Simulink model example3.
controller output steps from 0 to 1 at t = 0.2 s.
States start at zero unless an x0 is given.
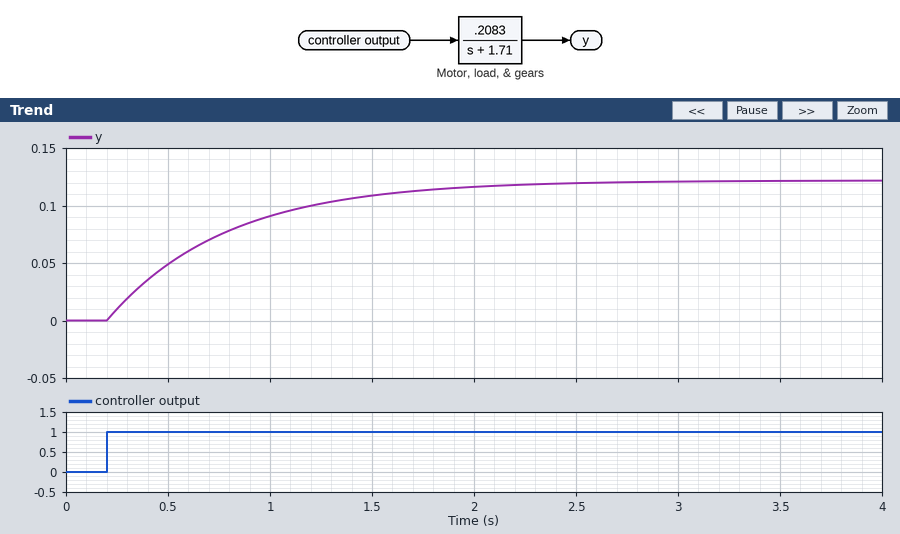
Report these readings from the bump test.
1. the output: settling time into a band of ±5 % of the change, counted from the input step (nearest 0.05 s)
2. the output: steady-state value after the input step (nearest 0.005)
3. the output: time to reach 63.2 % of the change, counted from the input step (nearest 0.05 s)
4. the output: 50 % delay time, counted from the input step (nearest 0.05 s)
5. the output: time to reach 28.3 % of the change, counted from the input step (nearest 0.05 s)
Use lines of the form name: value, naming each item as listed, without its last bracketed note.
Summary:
the output: settling time into a band of ±5 % of the change, counted from the input step: 1.75 s
the output: steady-state value after the input step: 0.120
the output: time to reach 63.2 % of the change, counted from the input step: 0.60 s
the output: 50 % delay time, counted from the input step: 0.40 s
the output: time to reach 28.3 % of the change, counted from the input step: 0.20 s
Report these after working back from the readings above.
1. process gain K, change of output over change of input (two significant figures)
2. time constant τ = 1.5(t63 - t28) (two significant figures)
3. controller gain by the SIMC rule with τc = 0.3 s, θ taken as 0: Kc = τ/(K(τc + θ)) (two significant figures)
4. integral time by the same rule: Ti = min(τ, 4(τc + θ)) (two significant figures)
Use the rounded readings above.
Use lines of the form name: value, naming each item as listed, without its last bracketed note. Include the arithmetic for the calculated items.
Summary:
process gain K, change of output over change of input: (0.12 - 0) / 1 = 0.12
time constant τ = 1.5(t63 - t28): 1.5 × (0.6 - 0.2) = 0.60 s
controller gain by the SIMC rule with τc = 0.3 s, θ taken as 0: Kc = τ/(K(τc + θ)): 0.6 / (0.12 × (0.3 + 0)) = 17
integral time by the same rule: Ti = min(τ, 4(τc + θ)): min(0.6, 4 × (0.3 + 0)) = 0.60 s
